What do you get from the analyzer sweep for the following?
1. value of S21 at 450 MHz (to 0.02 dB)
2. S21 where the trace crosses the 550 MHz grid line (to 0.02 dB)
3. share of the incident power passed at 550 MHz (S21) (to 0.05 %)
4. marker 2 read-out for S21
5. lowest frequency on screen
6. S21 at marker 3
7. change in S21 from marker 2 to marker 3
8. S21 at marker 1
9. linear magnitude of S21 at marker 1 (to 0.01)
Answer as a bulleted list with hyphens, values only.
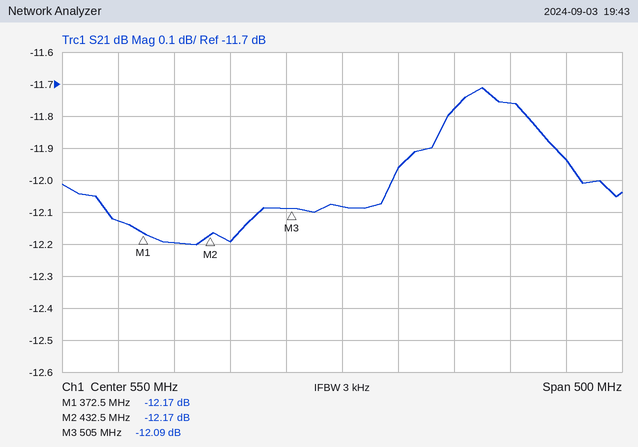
- -12.20 dB
- -12.08 dB
- 6.20 %
- -12.17 dB
- 300 MHz
- -12.09 dB
- 0.08 dB
- -12.17 dB
- 0.25
